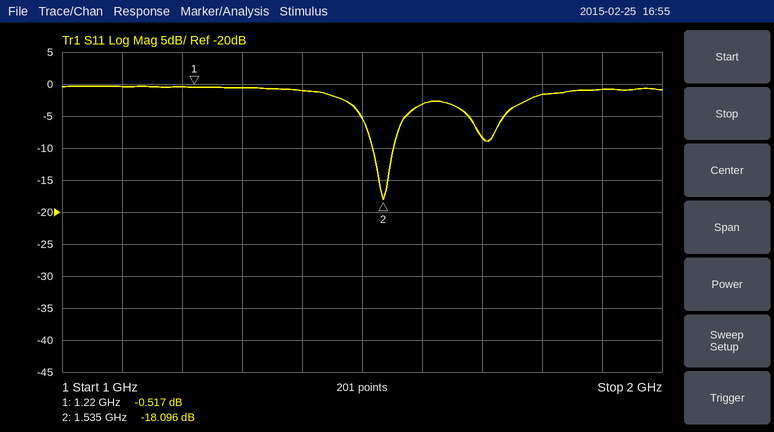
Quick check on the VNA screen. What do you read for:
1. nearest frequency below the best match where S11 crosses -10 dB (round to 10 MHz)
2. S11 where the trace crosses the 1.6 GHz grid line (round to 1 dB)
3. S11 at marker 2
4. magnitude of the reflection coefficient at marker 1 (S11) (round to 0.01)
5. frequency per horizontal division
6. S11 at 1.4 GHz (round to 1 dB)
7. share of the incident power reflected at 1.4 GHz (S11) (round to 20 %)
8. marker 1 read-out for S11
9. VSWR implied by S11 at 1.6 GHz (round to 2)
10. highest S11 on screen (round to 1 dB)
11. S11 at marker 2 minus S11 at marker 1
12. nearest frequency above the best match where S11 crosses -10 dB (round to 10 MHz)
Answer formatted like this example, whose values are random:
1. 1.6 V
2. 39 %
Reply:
1. 1.52 GHz
2. -3 dB
3. -18.096 dB
4. 0.94
5. 100 MHz
6. -1 dB
7. 80 %
8. -0.517 dB
9. 6
10. 0 dB
11. -17.579 dB
12. 1.55 GHz
